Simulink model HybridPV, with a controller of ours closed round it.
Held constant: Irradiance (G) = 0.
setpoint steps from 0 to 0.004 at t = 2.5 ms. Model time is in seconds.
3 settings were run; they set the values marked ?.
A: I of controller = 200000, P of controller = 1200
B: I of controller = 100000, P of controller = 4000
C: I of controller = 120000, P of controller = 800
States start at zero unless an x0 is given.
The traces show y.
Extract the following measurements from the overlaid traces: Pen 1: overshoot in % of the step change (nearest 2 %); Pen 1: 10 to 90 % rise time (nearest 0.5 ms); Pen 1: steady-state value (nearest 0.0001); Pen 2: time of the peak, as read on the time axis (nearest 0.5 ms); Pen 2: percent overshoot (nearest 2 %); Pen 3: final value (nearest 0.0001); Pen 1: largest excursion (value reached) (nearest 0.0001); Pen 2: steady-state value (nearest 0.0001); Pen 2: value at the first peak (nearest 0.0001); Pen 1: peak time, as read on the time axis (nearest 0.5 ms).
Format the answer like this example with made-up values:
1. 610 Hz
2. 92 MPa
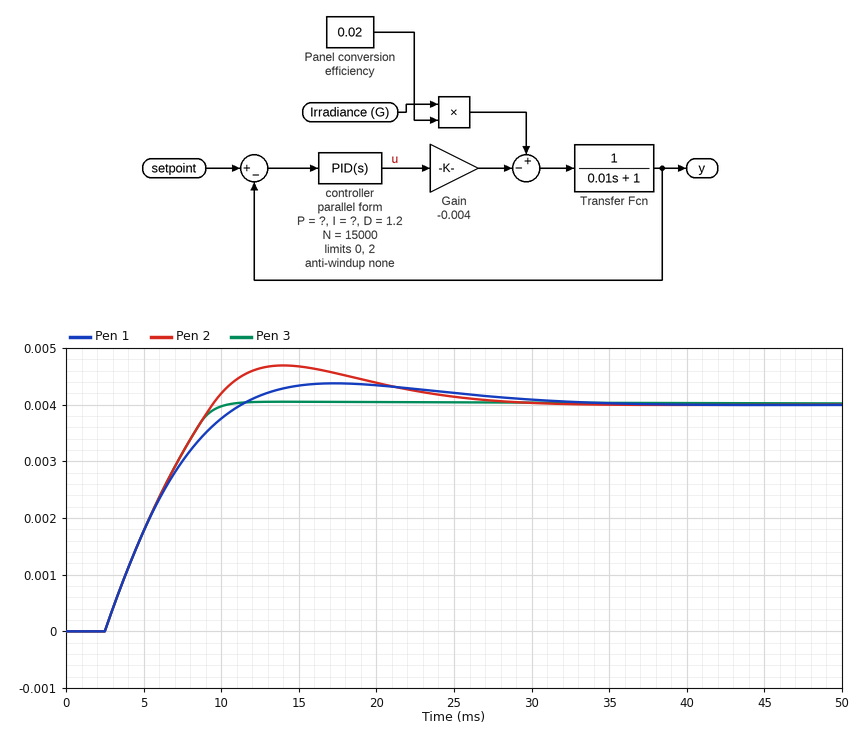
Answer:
1. 10 %
2. 6.5 ms
3. 0.0040
4. 14.0 ms
5. 18 %
6. 0.0040
7. 0.0044
8. 0.0040
9. 0.0047
10. 17.5 ms
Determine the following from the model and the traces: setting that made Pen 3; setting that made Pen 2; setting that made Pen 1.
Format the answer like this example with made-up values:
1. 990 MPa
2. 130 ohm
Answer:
1. B
2. A
3. C
